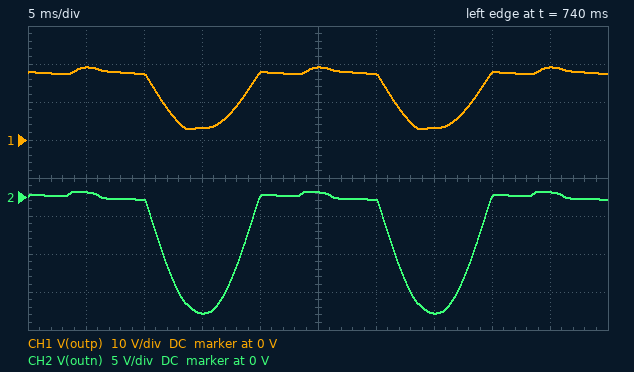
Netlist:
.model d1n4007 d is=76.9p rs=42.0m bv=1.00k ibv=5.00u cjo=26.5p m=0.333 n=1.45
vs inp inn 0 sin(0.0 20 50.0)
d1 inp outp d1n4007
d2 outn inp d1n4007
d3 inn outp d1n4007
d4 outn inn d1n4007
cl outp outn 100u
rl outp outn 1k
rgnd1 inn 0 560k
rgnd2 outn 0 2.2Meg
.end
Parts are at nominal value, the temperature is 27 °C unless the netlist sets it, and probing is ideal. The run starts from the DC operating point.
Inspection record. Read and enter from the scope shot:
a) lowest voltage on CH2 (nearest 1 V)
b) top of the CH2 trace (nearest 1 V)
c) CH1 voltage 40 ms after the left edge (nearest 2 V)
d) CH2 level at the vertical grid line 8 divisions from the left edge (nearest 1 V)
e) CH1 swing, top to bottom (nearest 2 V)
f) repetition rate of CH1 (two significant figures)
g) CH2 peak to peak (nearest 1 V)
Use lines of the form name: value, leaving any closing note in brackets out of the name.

lowest voltage on CH2: -15 V
top of the CH2 trace: 1 V
CH1 voltage 40 ms after the left edge: 18 V
CH2 level at the vertical grid line 8 divisions from the left edge: 0 V
CH1 swing, top to bottom: 16 V
repetition rate of CH1: 50 Hz
CH2 peak to peak: 16 V
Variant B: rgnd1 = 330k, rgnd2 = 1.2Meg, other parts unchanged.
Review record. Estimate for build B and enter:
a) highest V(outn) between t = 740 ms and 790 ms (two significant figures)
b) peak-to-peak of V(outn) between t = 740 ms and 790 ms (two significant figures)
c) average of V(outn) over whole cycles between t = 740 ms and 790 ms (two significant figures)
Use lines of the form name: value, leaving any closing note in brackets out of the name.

highest V(outn) between t = 740 ms and 790 ms: 650 mV
peak-to-peak of V(outn) between t = 740 ms and 790 ms: 16 V
average of V(outn) over whole cycles between t = 740 ms and 790 ms: -4.7 V
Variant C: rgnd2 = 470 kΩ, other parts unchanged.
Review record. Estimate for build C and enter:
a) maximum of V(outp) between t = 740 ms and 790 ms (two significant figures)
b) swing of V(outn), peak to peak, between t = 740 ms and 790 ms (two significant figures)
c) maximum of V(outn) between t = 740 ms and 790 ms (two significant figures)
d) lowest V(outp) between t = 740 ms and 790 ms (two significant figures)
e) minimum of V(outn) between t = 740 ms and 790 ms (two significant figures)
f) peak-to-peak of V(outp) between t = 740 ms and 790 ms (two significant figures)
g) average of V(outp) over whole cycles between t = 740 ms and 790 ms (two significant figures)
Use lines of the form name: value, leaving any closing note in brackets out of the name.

maximum of V(outp) between t = 740 ms and 790 ms: 19 V
swing of V(outn), peak to peak, between t = 740 ms and 790 ms: 9.2 V
maximum of V(outn) between t = 740 ms and 790 ms: 380 mV
lowest V(outp) between t = 740 ms and 790 ms: 8.9 V
minimum of V(outn) between t = 740 ms and 790 ms: -8.8 V
peak-to-peak of V(outp) between t = 740 ms and 790 ms: 9.9 V
average of V(outp) over whole cycles between t = 740 ms and 790 ms: 15 V
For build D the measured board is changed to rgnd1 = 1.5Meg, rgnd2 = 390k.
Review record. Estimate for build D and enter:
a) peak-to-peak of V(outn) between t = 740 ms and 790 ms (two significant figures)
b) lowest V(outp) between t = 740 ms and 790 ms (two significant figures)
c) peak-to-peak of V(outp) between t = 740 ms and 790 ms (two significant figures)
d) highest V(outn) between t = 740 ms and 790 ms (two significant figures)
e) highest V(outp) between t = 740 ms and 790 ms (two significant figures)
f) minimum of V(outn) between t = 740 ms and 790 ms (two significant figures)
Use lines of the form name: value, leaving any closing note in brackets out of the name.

peak-to-peak of V(outn) between t = 740 ms and 790 ms: 4.1 V
lowest V(outp) between t = 740 ms and 790 ms: 13 V
peak-to-peak of V(outp) between t = 740 ms and 790 ms: 5.3 V
highest V(outn) between t = 740 ms and 790 ms: 170 mV
highest V(outp) between t = 740 ms and 790 ms: 19 V
minimum of V(outn) between t = 740 ms and 790 ms: -4.0 V
